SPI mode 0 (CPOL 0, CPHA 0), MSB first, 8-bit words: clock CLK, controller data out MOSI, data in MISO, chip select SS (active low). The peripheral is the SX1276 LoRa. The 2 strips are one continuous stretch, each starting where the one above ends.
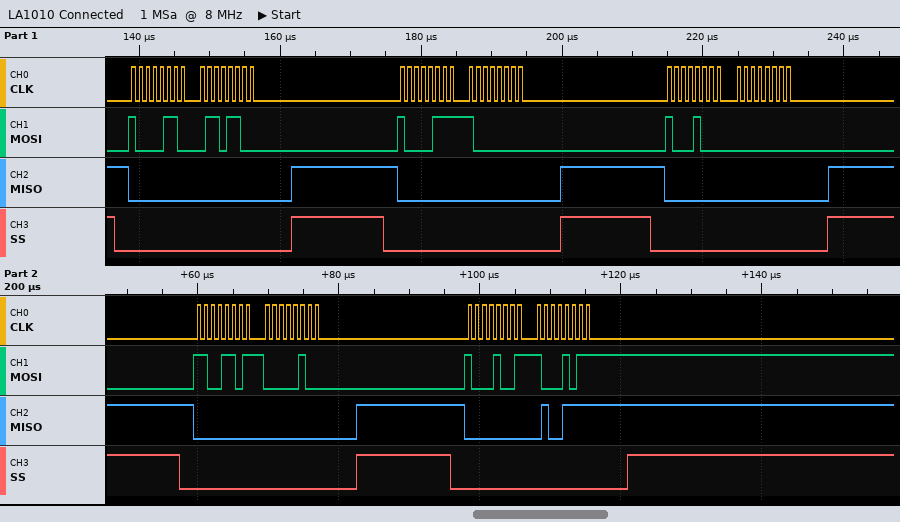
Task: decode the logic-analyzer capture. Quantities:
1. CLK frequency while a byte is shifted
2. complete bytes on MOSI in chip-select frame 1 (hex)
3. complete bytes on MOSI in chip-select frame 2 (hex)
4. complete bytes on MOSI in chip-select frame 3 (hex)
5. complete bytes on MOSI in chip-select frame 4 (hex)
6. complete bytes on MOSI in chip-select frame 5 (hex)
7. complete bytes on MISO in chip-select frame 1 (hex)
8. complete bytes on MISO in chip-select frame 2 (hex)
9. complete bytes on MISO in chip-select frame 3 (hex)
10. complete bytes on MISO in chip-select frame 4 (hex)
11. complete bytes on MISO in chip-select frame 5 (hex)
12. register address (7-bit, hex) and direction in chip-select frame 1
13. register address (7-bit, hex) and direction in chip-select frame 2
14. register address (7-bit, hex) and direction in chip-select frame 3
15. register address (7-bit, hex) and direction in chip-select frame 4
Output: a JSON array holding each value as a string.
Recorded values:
["1 MHz", "86 6C", "87 80", "88 00", "CD 04", "89 8B", "00 00", "00 00", "00 00", "00 00", "00 4F", "0x06 write", "0x07 write", "0x08 write", "0x4D write"]
